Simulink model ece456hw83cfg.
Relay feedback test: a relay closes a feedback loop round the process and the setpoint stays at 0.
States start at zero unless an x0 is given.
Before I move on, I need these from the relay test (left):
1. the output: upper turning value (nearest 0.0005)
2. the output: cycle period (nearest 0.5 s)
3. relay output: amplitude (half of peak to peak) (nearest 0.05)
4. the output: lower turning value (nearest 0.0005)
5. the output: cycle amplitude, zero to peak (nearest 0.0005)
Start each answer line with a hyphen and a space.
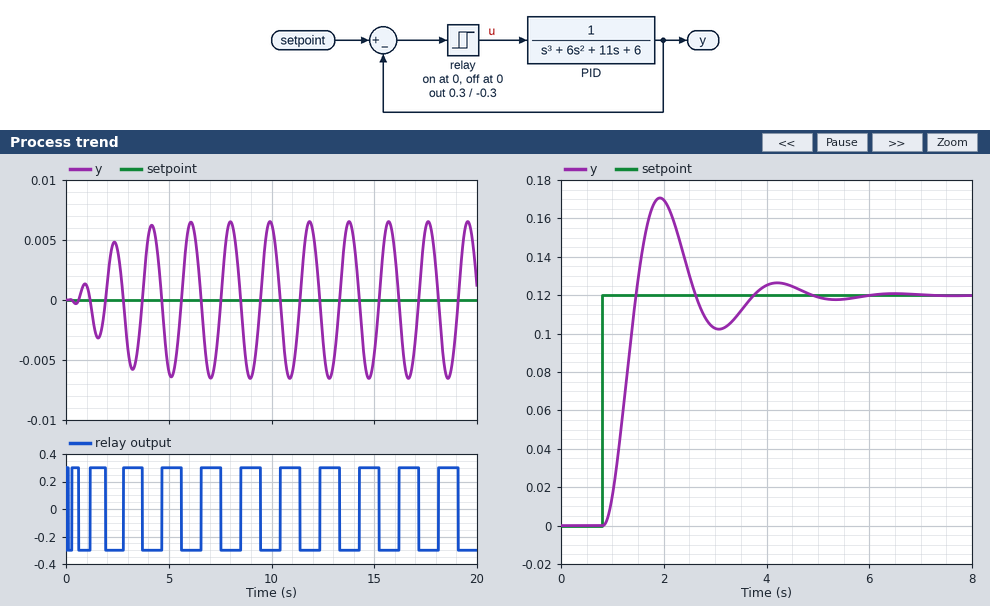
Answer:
- 0.0065
- 2.0 s
- 0.30
- -0.0065
- 0.0065
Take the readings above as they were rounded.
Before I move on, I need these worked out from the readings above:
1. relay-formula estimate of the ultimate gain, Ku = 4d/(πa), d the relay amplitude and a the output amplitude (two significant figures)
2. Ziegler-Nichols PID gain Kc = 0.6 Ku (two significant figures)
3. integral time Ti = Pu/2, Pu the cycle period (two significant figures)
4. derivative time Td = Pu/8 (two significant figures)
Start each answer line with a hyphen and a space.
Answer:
- 59
- 35
- 1.0 s
- 0.25 s
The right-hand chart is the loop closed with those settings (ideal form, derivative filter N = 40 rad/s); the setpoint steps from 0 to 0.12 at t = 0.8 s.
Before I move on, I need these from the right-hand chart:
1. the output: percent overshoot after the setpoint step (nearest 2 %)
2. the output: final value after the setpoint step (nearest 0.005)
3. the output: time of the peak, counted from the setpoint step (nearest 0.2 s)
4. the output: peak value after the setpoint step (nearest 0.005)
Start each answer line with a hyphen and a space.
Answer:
- 42 %
- 0.120
- 1.2 s
- 0.170
